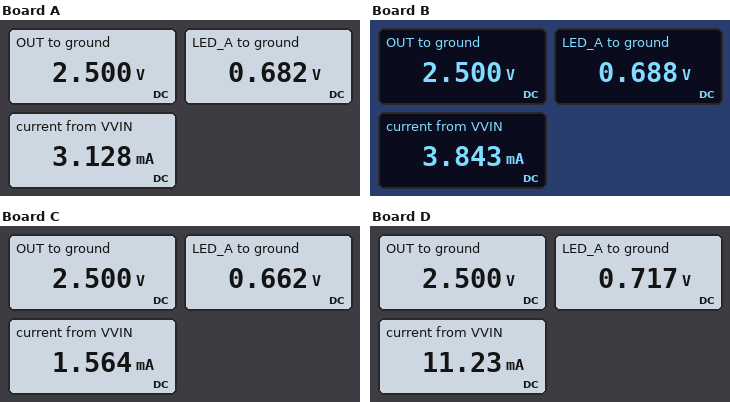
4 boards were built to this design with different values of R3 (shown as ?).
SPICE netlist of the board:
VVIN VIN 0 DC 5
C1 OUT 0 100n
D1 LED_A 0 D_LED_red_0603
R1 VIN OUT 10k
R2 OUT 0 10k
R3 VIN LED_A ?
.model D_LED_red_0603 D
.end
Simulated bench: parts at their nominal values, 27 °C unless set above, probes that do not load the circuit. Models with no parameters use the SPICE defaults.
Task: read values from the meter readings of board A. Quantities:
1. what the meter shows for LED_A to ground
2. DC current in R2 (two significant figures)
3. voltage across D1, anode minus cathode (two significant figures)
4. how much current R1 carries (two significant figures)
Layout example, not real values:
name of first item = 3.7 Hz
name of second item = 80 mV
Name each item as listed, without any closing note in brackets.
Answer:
what the meter shows for LED_A to ground = 0.682 V
DC current in R2 = 250 µA
voltage across D1, anode minus cathode = 680 mV
how much current R1 carries = 250 µA
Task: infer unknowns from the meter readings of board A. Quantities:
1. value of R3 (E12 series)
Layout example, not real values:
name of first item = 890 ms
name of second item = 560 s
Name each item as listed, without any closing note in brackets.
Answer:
value of R3 = 1.5 kΩ
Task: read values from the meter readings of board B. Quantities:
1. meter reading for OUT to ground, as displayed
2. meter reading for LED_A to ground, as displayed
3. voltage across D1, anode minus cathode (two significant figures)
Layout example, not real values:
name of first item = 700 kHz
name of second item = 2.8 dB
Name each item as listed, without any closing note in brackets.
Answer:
meter reading for OUT to ground, as displayed = 2.500 V
meter reading for LED_A to ground, as displayed = 0.688 V
voltage across D1, anode minus cathode = 690 mV
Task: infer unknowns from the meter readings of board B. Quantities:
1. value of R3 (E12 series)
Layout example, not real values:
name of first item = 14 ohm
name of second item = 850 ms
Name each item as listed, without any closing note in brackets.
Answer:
value of R3 = 1.2 kΩ
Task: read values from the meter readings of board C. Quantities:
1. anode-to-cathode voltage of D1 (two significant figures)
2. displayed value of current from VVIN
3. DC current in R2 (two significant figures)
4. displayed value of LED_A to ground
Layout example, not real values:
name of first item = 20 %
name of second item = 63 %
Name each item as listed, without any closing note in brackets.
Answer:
anode-to-cathode voltage of D1 = 660 mV
displayed value of current from VVIN = 1.564 mA
DC current in R2 = 250 µA
displayed value of LED_A to ground = 0.662 V
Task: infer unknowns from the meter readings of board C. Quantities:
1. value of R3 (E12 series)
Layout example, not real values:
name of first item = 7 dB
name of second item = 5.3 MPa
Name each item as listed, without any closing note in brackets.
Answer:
value of R3 = 3.3 kΩ
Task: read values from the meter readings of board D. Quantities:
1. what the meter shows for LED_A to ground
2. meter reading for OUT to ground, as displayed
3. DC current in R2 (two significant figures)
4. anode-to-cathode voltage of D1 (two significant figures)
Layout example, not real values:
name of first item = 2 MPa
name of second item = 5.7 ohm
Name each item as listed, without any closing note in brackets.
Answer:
what the meter shows for LED_A to ground = 0.717 V
meter reading for OUT to ground, as displayed = 2.500 V
DC current in R2 = 250 µA
anode-to-cathode voltage of D1 = 720 mV
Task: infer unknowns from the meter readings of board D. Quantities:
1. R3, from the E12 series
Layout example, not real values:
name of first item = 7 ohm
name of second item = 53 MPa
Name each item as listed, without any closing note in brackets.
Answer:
R3, from the E12 series = 390 Ω
